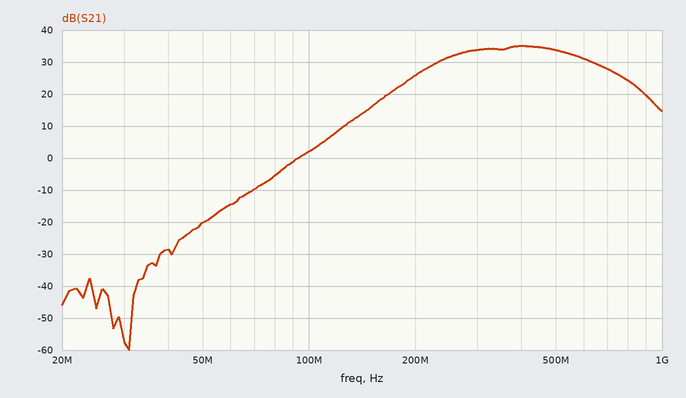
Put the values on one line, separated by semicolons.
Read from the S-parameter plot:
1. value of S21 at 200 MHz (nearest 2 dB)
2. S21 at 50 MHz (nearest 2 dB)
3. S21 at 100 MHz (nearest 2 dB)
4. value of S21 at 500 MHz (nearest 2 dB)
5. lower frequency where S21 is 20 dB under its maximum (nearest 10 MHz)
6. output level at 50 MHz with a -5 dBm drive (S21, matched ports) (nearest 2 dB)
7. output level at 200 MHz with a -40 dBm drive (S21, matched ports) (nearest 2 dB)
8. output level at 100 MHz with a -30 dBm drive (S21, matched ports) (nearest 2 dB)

26 dB; -20 dB; 2 dB; 34 dB; 150 MHz; -26 dBm; -14 dBm; -28 dBm
